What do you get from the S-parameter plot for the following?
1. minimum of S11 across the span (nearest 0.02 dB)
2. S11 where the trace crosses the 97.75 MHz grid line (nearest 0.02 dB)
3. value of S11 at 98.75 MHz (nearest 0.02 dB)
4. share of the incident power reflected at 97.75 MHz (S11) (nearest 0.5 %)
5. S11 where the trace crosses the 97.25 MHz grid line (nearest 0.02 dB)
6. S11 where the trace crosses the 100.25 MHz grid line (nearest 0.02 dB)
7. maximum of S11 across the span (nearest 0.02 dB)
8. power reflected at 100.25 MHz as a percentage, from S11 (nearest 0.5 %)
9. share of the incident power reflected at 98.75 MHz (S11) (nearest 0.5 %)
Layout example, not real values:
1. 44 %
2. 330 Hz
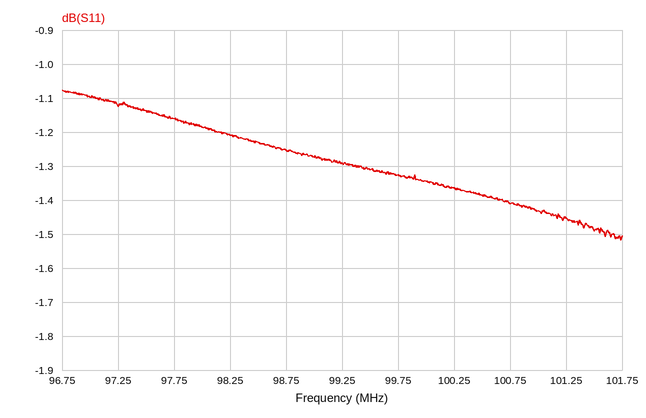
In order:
1. -1.52 dB
2. -1.16 dB
3. -1.26 dB
4. 76.5 %
5. -1.12 dB
6. -1.36 dB
7. -1.08 dB
8. 73.0 %
9. 75.0 %
